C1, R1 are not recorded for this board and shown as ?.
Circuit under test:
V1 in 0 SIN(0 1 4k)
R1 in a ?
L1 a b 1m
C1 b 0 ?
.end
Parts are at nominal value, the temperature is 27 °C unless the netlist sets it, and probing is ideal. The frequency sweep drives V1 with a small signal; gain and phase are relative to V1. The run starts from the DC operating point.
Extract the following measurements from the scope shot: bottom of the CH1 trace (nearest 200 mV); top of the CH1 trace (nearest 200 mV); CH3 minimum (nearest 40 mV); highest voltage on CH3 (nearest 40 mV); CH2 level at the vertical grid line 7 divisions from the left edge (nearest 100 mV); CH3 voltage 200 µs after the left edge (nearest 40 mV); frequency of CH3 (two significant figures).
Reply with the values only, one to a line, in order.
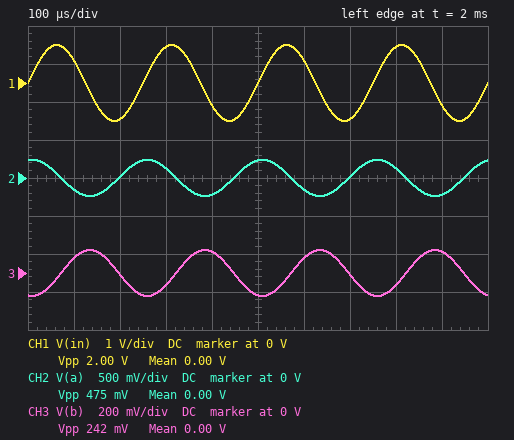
-1.0 V
1.0 V
-120 mV
120 mV
0 V
0 V
4.0 kHz
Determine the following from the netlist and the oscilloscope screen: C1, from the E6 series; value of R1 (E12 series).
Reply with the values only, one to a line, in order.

4.7 µF
68 Ω
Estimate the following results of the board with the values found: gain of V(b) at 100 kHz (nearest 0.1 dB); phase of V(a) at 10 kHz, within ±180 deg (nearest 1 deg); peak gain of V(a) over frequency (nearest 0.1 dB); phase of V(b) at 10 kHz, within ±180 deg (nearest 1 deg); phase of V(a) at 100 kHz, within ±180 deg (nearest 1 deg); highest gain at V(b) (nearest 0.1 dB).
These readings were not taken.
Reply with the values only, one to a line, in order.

-65.4 dB
49 deg
0 dB
-131 deg
6 deg
0 dB
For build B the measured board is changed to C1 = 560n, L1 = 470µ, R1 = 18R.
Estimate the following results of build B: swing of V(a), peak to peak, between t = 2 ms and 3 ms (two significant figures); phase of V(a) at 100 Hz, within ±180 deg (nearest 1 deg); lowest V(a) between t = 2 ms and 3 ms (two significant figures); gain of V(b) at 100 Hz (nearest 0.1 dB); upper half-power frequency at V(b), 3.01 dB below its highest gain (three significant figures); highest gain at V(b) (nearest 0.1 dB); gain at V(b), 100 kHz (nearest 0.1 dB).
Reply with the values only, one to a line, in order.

1.9 V
0 deg
-960 mV
0 dB
11.6 kHz
4.6 dB
-40.3 dB
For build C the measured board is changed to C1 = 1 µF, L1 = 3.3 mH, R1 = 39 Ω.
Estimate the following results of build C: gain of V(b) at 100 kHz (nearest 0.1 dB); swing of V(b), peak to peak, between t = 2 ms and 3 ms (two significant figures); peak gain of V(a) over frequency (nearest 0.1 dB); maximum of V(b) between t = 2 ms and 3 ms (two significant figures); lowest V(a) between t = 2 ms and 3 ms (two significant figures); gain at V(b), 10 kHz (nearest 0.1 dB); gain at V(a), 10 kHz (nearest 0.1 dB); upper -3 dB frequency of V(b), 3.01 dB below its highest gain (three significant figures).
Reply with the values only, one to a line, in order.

-62.3 dB
1.4 V
0 dB
680 mV
-740 mV
-21.8 dB
-0.2 dB
3.29 kHz
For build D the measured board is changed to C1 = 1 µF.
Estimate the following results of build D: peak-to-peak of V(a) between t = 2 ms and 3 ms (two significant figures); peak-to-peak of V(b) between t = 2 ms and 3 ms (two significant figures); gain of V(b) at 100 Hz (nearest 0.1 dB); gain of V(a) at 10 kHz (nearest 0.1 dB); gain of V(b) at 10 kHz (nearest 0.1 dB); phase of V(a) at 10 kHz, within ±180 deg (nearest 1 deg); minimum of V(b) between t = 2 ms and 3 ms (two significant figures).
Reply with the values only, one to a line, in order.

420 mV
1.1 V
0 dB
-4.9 dB
-14.3 dB
55 deg
-570 mV
